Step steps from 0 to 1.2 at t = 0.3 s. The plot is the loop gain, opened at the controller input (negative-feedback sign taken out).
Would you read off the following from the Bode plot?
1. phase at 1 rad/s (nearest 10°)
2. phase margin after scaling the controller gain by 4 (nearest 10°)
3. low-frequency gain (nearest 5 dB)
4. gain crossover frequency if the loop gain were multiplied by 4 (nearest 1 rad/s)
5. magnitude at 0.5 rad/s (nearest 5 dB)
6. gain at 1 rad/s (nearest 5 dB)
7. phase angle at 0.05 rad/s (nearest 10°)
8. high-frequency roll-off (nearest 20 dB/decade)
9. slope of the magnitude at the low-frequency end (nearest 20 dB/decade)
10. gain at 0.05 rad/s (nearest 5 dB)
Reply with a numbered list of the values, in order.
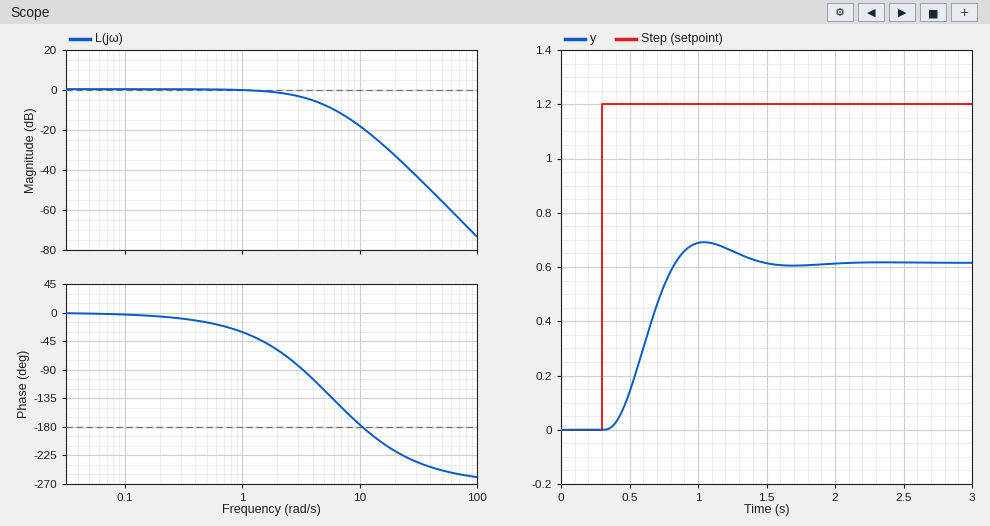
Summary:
1. -30°
2. 30°
3. 0 dB
4. 7 rad/s
5. 0 dB
6. 0 dB
7. 0°
8. -60 dB/decade
9. 0 dB/decade
10. 0 dB
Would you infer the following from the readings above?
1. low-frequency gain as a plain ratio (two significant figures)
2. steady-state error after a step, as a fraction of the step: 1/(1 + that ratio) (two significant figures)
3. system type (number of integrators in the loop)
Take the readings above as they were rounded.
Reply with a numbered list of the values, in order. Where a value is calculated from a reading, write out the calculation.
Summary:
1. 10^(0 / 20) = 1.0
2. 1 / (1 + 1) = 0.50
3. 0
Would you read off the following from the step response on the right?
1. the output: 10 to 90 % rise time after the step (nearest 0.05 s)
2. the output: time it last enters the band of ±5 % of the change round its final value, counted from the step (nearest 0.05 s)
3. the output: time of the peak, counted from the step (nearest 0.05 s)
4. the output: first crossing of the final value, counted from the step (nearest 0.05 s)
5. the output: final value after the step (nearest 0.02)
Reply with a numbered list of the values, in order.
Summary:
1. 0.35 s
2. 1.00 s
3. 0.75 s
4. 0.55 s
5. 0.62
